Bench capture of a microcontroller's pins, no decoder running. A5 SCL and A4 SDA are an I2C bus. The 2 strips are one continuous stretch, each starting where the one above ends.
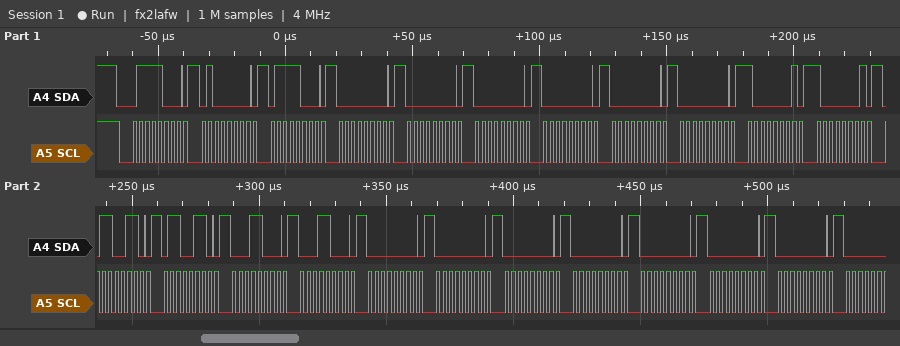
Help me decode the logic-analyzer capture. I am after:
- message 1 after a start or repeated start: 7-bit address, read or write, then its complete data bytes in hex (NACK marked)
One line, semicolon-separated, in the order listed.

0x3C write: 40 78 00 00 00 00 00 00 81 81 66 66 18 18 00 00 00 00 00 00 00
